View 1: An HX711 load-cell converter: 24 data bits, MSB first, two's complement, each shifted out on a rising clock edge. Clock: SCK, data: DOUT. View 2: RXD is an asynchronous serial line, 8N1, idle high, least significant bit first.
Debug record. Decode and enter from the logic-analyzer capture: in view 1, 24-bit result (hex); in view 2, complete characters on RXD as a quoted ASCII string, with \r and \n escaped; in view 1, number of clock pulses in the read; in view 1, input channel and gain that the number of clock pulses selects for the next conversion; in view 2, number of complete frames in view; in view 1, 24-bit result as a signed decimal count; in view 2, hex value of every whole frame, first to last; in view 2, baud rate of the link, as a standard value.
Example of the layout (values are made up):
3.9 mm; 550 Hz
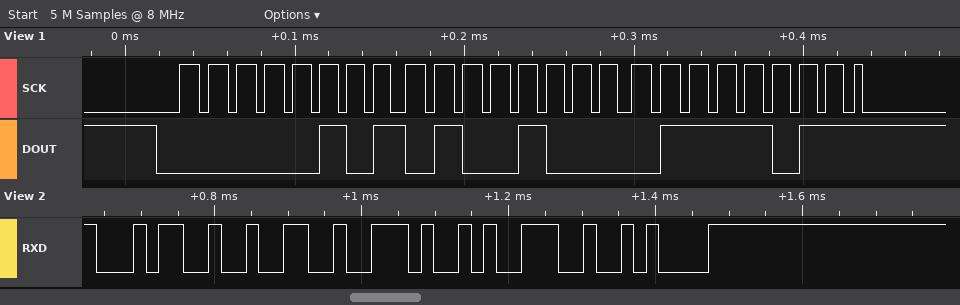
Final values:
0x05487B; "42.9\n"; 25; channel A, gain 128; 5; 346235; 34 32 2E 39 0A; 57600 baud
